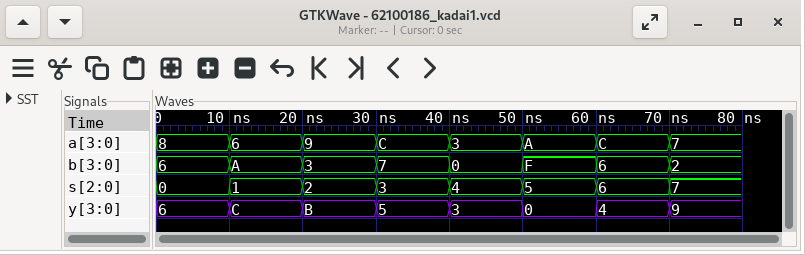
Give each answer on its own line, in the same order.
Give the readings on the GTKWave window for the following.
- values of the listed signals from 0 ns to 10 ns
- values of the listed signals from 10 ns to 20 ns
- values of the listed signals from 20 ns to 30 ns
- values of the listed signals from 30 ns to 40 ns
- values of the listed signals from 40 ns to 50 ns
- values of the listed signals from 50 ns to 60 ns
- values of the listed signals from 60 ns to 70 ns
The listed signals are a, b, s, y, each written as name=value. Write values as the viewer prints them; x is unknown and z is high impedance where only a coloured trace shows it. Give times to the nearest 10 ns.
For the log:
a=8, b=6, s=0, y=6
a=6, b=A, s=1, y=C
a=9, b=3, s=2, y=B
a=C, b=7, s=3, y=5
a=3, b=0, s=4, y=3
a=A, b=F, s=5, y=0
a=C, b=6, s=6, y=4
